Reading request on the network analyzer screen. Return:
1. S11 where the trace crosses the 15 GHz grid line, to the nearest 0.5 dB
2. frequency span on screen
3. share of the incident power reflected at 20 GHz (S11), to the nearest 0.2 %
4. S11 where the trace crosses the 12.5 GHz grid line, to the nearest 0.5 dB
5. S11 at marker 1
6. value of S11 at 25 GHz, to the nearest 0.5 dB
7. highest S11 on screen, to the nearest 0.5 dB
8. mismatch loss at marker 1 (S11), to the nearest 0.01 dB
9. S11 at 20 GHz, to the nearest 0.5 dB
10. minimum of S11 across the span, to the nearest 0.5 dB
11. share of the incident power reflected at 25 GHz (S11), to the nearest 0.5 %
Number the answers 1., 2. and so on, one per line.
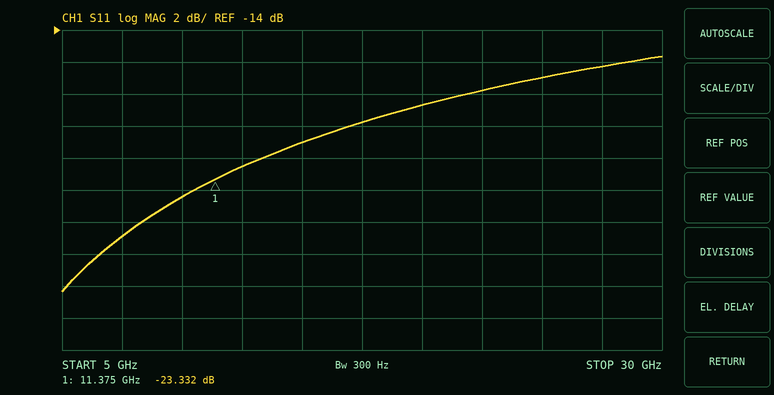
1. -21.0 dB
2. 25 GHz
3. 1.4 %
4. -22.5 dB
5. -23.332 dB
6. -17.0 dB
7. -15.5 dB
8. 0.02 dB
9. -18.5 dB
10. -30.5 dB
11. 2.0 %
